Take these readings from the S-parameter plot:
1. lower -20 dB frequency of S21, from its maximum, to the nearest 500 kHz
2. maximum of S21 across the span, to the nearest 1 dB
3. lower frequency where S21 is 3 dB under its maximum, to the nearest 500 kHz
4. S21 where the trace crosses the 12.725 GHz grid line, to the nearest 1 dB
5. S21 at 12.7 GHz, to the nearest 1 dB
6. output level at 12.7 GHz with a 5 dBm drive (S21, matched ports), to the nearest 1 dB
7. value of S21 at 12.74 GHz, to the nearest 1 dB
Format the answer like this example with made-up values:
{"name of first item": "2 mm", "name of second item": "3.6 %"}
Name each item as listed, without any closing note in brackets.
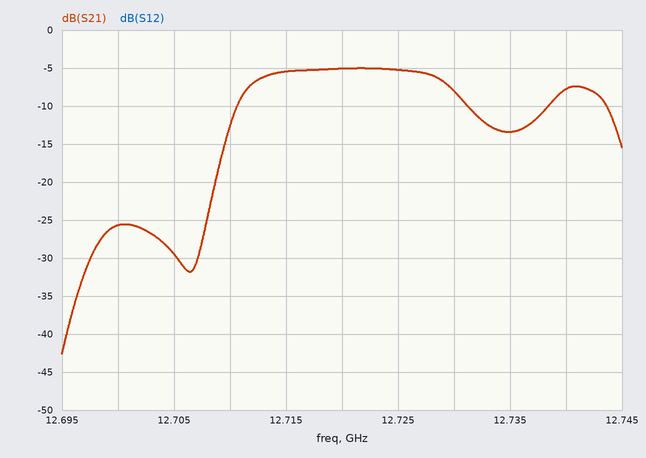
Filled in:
{"lower -20 dB frequency of S21, from its maximum, to the nearest 500 kHz": "12.7080 GHz", "maximum of S21 across the span, to the nearest 1 dB": "-5 dB", "lower frequency where S21 is 3 dB under its maximum, to the nearest 500 kHz": "12.7115 GHz", "S21 where the trace crosses the 12.725 GHz grid line, to the nearest 1 dB": "-5 dB", "S21 at 12.7 GHz, to the nearest 1 dB": "-26 dB", "output level at 12.7 GHz with a 5 dBm drive (S21, matched ports), to the nearest 1 dB": "-21 dBm", "value of S21 at 12.74 GHz, to the nearest 1 dB": "-8 dB"}
